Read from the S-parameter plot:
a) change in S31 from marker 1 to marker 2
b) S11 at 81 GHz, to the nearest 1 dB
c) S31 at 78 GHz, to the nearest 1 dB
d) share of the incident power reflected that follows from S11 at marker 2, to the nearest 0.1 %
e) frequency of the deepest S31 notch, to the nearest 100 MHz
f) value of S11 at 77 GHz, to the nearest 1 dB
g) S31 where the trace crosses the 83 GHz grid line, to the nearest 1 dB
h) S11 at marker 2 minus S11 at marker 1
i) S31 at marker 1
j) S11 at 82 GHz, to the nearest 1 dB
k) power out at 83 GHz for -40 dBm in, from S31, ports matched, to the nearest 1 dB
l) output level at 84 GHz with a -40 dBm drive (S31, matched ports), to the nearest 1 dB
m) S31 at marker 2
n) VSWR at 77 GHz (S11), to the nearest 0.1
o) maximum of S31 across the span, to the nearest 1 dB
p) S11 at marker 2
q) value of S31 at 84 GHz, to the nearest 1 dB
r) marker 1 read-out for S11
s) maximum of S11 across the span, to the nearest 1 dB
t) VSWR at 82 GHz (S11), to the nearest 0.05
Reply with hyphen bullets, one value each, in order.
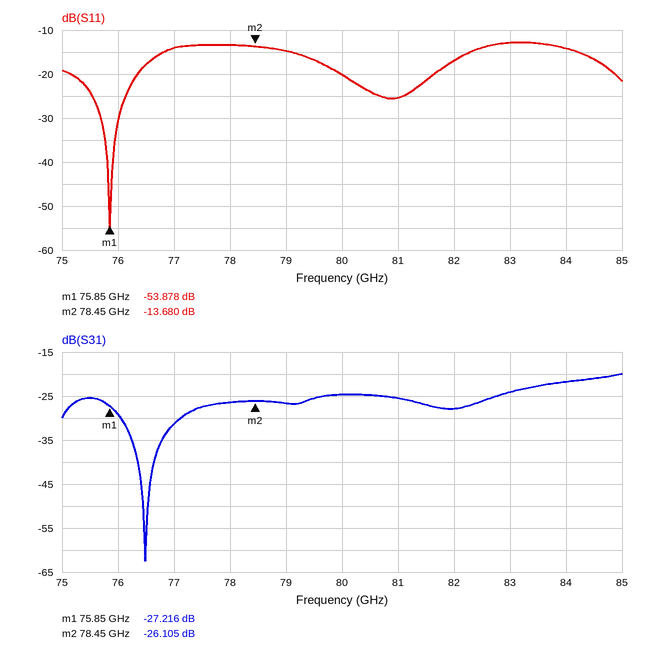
- 1.111 dB
- -25 dB
- -26 dB
- 4.3 %
- 76.5 GHz
- -14 dB
- -24 dB
- 40.198 dB
- -27.216 dB
- -17 dB
- -64 dBm
- -62 dBm
- -26.105 dB
- 1.5
- -20 dB
- -13.680 dB
- -22 dB
- -53.878 dB
- -13 dB
- 1.35
